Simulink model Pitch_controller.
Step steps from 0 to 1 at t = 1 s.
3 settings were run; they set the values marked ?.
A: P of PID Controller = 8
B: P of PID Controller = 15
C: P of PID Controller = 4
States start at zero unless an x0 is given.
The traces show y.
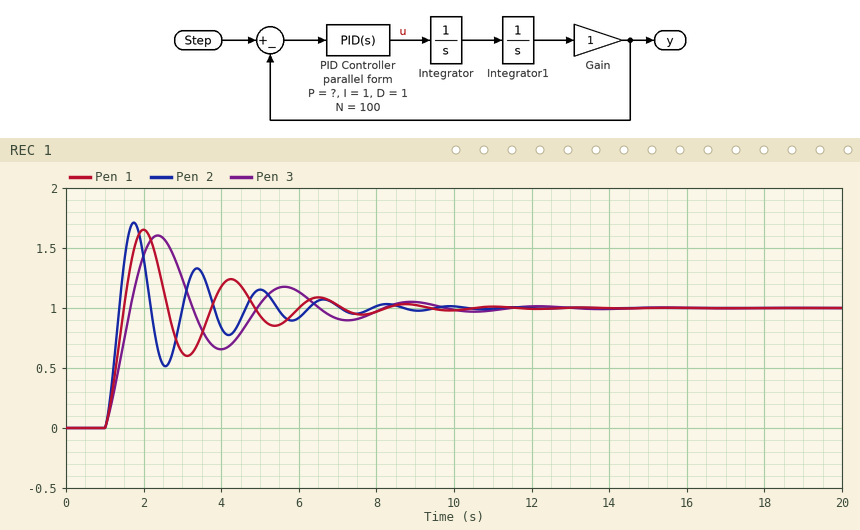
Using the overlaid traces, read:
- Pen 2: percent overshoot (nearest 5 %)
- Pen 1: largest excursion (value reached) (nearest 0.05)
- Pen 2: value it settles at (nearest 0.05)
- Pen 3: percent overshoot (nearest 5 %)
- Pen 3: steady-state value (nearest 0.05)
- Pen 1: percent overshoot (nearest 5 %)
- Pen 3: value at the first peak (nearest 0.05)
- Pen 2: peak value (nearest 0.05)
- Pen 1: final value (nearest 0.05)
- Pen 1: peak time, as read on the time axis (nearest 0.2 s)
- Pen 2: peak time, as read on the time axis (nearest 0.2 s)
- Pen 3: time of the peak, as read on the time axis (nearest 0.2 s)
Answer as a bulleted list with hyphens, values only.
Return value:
- 70 %
- 1.65
- 1.00
- 60 %
- 1.00
- 65 %
- 1.60
- 1.70
- 1.00
- 2.0 s
- 1.8 s
- 2.4 s
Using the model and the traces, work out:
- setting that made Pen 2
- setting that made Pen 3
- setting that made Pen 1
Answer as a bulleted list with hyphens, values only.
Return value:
- B
- C
- A
